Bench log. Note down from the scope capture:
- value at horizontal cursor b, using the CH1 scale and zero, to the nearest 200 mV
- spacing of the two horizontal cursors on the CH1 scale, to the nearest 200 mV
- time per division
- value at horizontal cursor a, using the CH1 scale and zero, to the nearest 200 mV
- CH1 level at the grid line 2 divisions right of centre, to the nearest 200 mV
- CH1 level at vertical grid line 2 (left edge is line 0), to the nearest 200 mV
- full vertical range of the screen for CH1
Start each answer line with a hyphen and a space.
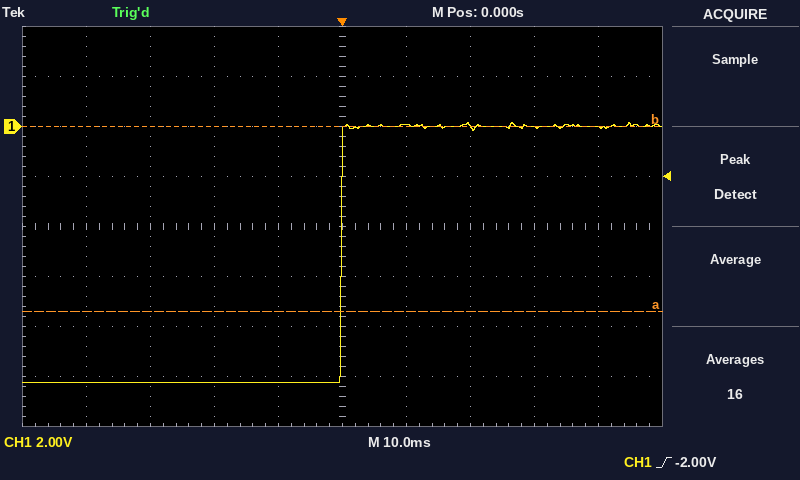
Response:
- 0.0 V
- 7.4 V
- 10 ms
- -7.4 V
- 0.0 V
- -10.2 V
- 16 V
